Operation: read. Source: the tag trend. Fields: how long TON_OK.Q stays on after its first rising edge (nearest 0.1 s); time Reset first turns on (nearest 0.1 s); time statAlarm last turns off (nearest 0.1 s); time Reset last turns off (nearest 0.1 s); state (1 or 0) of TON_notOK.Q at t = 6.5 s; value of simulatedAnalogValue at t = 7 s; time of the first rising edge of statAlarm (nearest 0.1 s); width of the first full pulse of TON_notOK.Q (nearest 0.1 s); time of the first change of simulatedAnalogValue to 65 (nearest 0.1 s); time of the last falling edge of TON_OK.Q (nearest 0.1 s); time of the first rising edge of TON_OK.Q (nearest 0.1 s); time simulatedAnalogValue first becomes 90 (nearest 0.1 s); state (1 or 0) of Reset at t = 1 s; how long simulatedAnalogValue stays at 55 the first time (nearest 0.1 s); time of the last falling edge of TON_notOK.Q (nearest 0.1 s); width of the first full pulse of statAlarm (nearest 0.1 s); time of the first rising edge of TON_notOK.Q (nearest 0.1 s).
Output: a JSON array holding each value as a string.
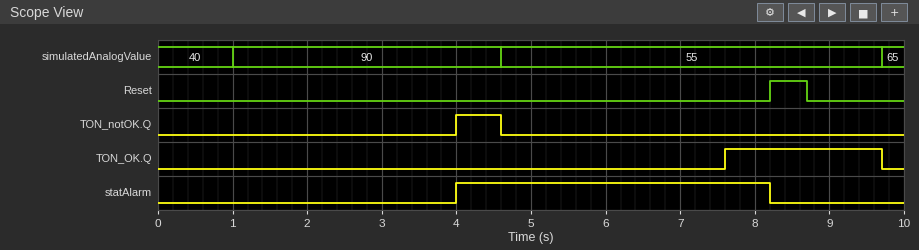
["2.1 s", "8.2 s", "8.2 s", "8.7 s", "0", "55", "4.0 s", "0.6 s", "9.7 s", "9.7 s", "7.6 s", "1.0 s", "0", "5.1 s", "4.6 s", "4.2 s", "4.0 s"]
